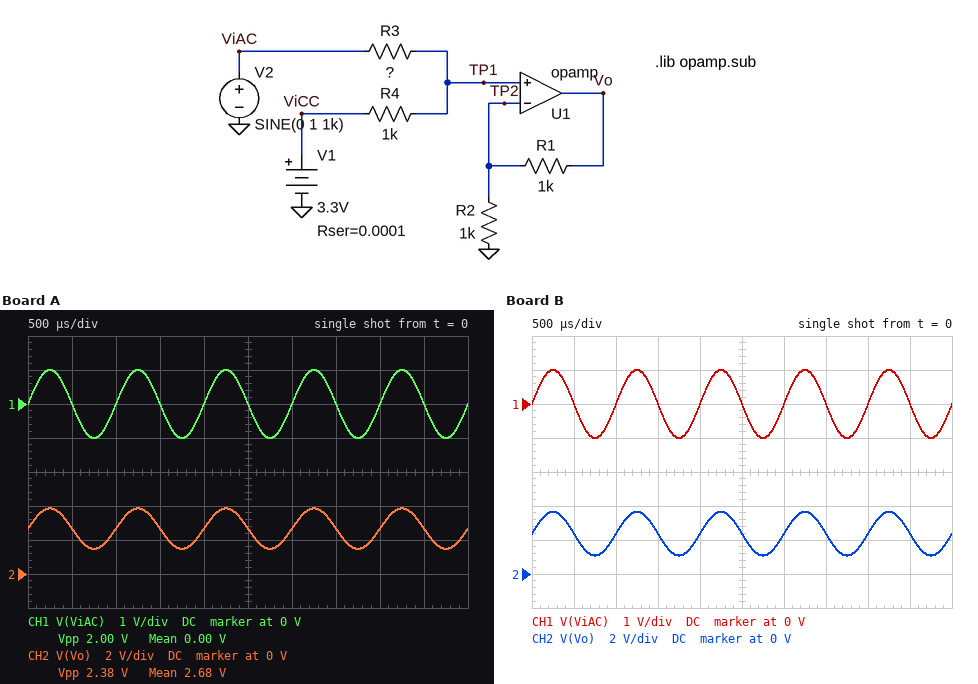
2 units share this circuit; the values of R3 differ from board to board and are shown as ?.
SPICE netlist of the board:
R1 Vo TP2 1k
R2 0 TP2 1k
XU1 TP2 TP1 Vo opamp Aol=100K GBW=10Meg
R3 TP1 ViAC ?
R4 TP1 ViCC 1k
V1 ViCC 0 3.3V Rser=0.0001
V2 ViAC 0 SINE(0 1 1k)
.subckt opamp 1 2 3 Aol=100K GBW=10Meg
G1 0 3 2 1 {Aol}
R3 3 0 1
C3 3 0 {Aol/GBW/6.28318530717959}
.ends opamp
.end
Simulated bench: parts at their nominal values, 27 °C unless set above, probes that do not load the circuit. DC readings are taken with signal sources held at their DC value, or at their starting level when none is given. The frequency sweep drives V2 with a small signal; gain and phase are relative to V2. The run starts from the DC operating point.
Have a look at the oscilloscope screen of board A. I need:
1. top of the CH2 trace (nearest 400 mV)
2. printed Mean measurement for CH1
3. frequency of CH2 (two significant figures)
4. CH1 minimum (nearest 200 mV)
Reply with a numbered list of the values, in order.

1. 4.0 V
2. 0.00 V
3. 1.0 kHz
4. -1.0 V
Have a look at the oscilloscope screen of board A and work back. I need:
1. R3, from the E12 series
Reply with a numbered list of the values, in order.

1. 680 Ω
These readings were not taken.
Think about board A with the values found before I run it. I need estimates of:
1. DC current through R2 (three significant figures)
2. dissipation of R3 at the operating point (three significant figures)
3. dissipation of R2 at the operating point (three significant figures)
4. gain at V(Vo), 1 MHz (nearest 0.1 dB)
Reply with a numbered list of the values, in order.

1. 1.34 mA
2. 2.62 mW
3. 1.78 mW
4. 1.3 dB
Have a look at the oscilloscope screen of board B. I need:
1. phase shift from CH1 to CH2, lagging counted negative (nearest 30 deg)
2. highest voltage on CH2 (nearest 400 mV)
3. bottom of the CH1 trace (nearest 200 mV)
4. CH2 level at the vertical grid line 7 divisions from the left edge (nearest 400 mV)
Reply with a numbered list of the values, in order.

1. 0 deg
2. 3.6 V
3. -1.0 V
4. 2.4 V
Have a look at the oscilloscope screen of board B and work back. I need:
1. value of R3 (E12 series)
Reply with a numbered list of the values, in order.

1. 560 Ω
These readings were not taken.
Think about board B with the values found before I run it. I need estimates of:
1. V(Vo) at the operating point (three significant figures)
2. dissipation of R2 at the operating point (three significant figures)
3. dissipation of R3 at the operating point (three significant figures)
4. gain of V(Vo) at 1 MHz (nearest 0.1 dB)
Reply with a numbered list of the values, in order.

1. 2.37 V
2. 1.40 mW
3. 2.51 mW
4. 2.0 dB
